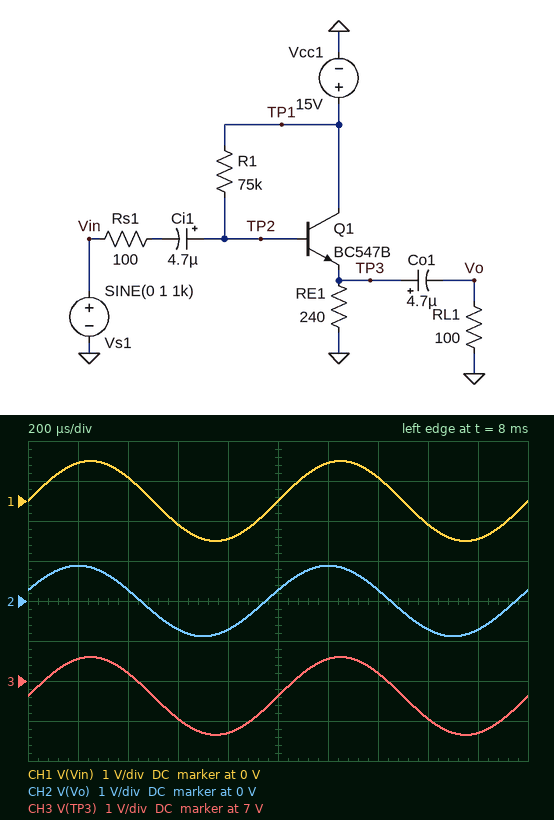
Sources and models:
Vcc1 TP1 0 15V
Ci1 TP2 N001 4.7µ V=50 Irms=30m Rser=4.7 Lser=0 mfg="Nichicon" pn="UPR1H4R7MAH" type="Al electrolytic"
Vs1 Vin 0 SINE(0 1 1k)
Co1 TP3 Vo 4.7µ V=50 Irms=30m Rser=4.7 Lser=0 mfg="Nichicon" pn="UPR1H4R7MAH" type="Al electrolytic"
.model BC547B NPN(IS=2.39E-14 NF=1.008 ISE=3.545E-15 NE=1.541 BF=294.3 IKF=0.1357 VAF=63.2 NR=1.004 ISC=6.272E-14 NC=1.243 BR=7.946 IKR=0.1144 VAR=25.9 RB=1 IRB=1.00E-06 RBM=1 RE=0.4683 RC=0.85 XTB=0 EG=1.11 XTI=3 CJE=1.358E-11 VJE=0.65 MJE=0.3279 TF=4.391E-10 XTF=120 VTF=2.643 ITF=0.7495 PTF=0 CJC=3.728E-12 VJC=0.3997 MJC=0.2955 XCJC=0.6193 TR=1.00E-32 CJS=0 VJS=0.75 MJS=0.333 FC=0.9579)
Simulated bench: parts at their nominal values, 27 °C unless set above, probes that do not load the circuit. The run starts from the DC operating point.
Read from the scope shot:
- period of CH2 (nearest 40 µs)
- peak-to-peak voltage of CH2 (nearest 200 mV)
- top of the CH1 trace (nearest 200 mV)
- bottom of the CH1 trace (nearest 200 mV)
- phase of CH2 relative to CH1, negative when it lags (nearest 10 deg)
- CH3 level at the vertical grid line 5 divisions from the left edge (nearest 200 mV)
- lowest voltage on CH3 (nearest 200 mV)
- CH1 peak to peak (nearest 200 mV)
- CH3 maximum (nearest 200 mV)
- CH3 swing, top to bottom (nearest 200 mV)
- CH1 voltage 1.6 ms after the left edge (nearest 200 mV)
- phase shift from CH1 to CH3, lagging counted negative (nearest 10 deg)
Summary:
1.00 ms
1.8 V
1.0 V
-1.0 V
20 deg
6.6 V
5.6 V
2.0 V
7.6 V
2.0 V
-600 mV
0 deg
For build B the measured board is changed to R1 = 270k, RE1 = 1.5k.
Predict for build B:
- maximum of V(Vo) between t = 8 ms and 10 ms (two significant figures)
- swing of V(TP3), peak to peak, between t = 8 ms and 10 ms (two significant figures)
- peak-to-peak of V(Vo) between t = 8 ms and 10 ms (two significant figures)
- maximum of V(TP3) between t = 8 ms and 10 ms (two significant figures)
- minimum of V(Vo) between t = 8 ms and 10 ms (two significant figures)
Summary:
800 mV
1.6 V
1.4 V
9.9 V
-570 mV
